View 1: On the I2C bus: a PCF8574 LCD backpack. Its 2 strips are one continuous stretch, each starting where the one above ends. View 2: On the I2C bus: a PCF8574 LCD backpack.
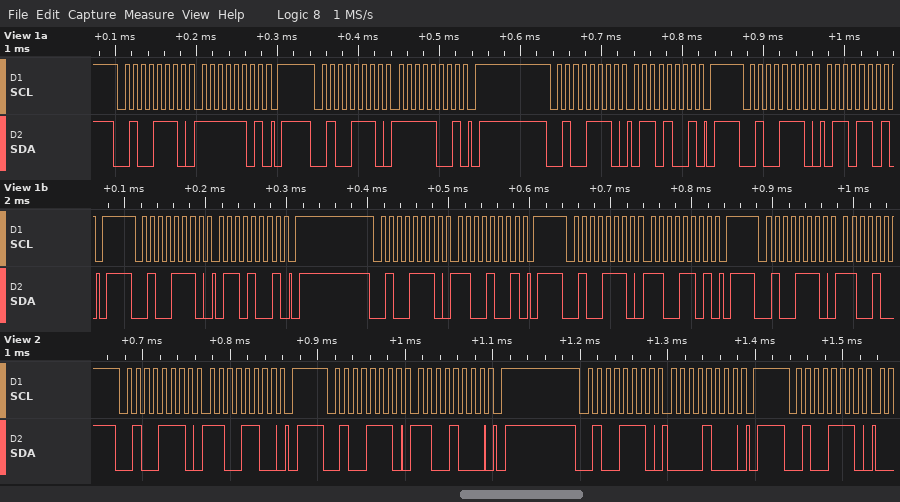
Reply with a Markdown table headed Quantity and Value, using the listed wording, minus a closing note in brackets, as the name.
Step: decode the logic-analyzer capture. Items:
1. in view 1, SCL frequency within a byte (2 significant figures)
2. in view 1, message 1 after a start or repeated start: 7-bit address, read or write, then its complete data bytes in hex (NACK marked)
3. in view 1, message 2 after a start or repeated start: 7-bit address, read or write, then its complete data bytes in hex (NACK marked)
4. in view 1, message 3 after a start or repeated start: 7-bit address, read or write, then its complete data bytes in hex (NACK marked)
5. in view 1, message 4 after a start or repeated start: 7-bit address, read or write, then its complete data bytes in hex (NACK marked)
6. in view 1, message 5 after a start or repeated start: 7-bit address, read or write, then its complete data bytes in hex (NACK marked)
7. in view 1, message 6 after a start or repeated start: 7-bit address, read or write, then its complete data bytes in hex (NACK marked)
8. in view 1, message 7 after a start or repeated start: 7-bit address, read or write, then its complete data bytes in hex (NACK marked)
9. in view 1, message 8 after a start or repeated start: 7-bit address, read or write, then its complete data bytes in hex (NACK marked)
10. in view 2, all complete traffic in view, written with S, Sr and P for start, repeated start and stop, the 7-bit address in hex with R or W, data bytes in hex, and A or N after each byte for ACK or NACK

| Quantity | Value |
|---|---|
| in view 1, SCL frequency within a byte | 100 kHz |
| in view 1, message 1 after a start or repeated start: 7-bit address, read or write, then its complete data bytes in hex | 0x27 write: FD |
| in view 1, message 2 after a start or repeated start: 7-bit address, read or write, then its complete data bytes in hex | 0x27 write: F9 |
| in view 1, message 3 after a start or repeated start: 7-bit address, read or write, then its complete data bytes in hex | 0x27 write: 69 |
| in view 1, message 4 after a start or repeated start: 7-bit address, read or write, then its complete data bytes in hex | 0x27 write: 6D |
| in view 1, message 5 after a start or repeated start: 7-bit address, read or write, then its complete data bytes in hex | 0x27 write: 69 |
| in view 1, message 6 after a start or repeated start: 7-bit address, read or write, then its complete data bytes in hex | 0x27 write: C9 |
| in view 1, message 7 after a start or repeated start: 7-bit address, read or write, then its complete data bytes in hex | 0x27 write: CD |
| in view 1, message 8 after a start or repeated start: 7-bit address, read or write, then its complete data bytes in hex | 0x27 write |
| in view 2, all complete traffic in view, written with S, Sr and P for start, repeated start and stop, the 7-bit address in hex with R or W, data bytes in hex, and A or N after each byte for ACK or NACK | S 27W A CC A P S 27W A C8 A P S 27W A 08 A P S 27W A |
